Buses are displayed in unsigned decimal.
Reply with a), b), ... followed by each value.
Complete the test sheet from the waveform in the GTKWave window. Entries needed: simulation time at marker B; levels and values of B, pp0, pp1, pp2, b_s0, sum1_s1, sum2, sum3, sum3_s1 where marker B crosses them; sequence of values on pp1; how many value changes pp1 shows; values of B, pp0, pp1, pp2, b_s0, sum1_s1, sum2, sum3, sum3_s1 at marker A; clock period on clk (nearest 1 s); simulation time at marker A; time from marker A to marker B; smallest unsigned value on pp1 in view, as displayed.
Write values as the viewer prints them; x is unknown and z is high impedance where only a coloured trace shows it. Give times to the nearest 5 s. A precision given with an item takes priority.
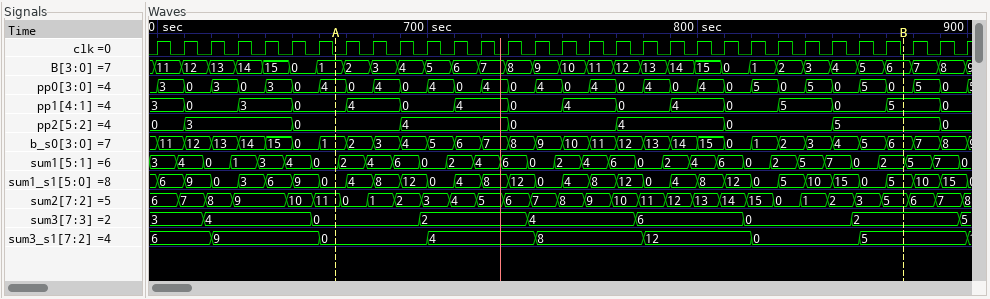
a) 875 s
b) B=6, pp0=0, pp1=5, pp2=5, b_s0=6, sum1_s1=5, sum2=5, sum3=2, sum3_s1=5
c) 3, 0, 3, 0, 4, 0, 4, 0, 4, 0, 4, 0, 5, 0, 5, 0
d) 15
e) B=1, pp0=4, pp1=0, pp2=0, b_s0=1, sum1_s1=0, sum2=11, sum3=0, sum3_s1=0
f) 10 s
g) 665 s
h) 210 s
i) 0
